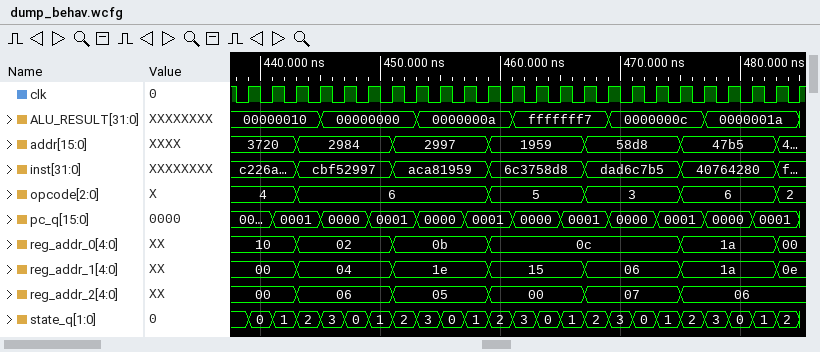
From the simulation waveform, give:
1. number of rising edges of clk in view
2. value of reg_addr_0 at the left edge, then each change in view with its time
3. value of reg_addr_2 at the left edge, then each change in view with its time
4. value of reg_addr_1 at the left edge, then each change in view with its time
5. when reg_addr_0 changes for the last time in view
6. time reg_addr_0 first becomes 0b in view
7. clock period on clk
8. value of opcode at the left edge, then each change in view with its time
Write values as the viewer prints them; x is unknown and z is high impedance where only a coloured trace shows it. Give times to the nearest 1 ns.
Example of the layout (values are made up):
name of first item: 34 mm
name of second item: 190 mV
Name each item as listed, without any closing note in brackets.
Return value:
number of rising edges of clk in view: 24
value of reg_addr_0 at the left edge, then each change in view with its time: 10, 02 at 443 ns, 0b at 451 ns, 0c at 459 ns, 1a at 475 ns, 00 at 483 ns
value of reg_addr_2 at the left edge, then each change in view with its time: 00, 06 at 443 ns, 05 at 451 ns, 00 at 459 ns, 07 at 467 ns, 06 at 475 ns
value of reg_addr_1 at the left edge, then each change in view with its time: 00, 04 at 443 ns, 1e at 451 ns, 15 at 459 ns, 06 at 467 ns, 1a at 475 ns, 0e at 483 ns
when reg_addr_0 changes for the last time in view: 483 ns
time reg_addr_0 first becomes 0b in view: 451 ns
clock period on clk: 2 ns
value of opcode at the left edge, then each change in view with its time: 4, 6 at 443 ns, 5 at 459 ns, 3 at 467 ns, 6 at 475 ns, 2 at 483 ns
